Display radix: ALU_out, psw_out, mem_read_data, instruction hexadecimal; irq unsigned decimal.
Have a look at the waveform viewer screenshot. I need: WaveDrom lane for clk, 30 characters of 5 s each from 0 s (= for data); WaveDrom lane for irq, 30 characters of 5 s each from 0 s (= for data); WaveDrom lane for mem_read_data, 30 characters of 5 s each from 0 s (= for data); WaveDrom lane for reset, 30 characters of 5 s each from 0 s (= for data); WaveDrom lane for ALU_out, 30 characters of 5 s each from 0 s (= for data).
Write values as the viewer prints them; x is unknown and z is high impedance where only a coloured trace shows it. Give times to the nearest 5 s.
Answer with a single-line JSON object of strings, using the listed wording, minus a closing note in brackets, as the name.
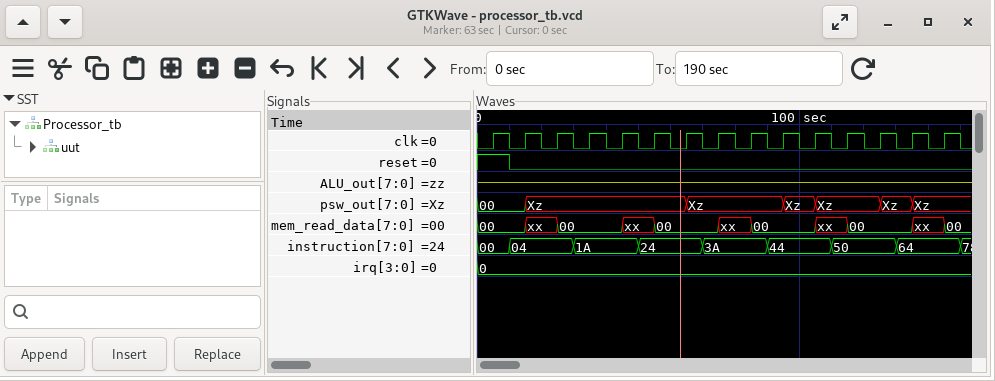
{"WaveDrom lane for clk, 30 characters of 5 s each from 0 s": "{name: 'clk', wave: '010101010101010101010101010101'}", "WaveDrom lane for irq, 30 characters of 5 s each from 0 s": "{name: 'irq', wave: '=.............................', data: '0'}", "WaveDrom lane for mem_read_data, 30 characters of 5 s each from 0 s": "{name: 'mem_read_data', wave: '=..x.=...x.=...x.=...x.=...x.=', data: '00 00 00 00 00 00'}", "WaveDrom lane for reset, 30 characters of 5 s each from 0 s": "{name: 'reset', wave: '1.0...........................'}", "WaveDrom lane for ALU_out, 30 characters of 5 s each from 0 s": "{name: 'ALU_out', wave: 'z.............................'}"}
